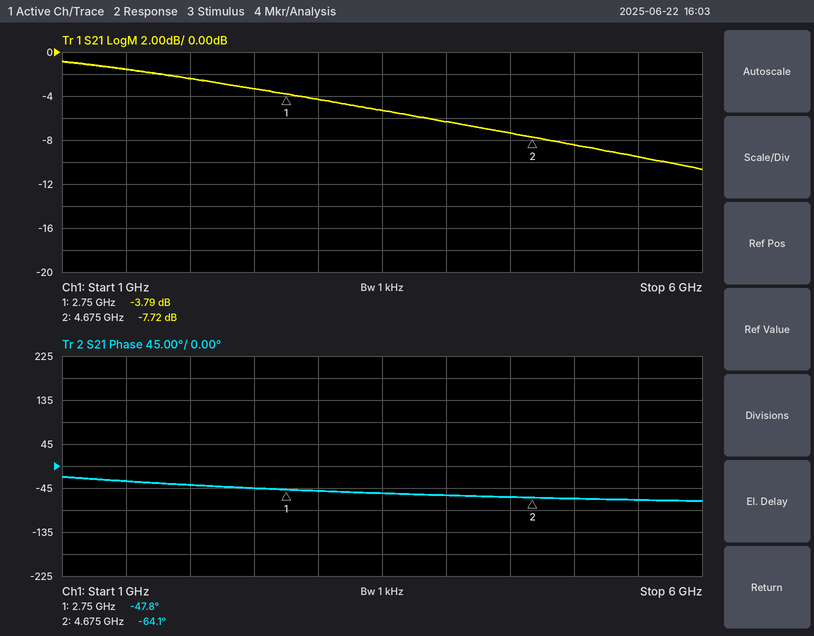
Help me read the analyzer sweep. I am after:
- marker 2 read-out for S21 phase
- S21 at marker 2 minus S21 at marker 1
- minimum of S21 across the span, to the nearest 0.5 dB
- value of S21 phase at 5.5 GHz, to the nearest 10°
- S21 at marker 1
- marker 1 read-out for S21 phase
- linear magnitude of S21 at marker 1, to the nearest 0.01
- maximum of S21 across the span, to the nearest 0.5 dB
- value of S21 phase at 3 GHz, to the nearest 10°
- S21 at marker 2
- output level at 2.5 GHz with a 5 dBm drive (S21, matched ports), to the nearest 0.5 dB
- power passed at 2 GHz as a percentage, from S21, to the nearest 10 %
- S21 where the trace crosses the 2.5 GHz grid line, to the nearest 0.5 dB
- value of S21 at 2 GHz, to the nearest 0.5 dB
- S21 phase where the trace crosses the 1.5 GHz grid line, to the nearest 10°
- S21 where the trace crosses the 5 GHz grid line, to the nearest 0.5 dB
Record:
-64.1°
-3.93 dB
-10.5 dB
-70°
-3.79 dB
-47.8°
0.65
-1.0 dB
-50°
-7.72 dB
1.5 dBm
60 %
-3.5 dB
-2.5 dB
-30°
-8.5 dB
